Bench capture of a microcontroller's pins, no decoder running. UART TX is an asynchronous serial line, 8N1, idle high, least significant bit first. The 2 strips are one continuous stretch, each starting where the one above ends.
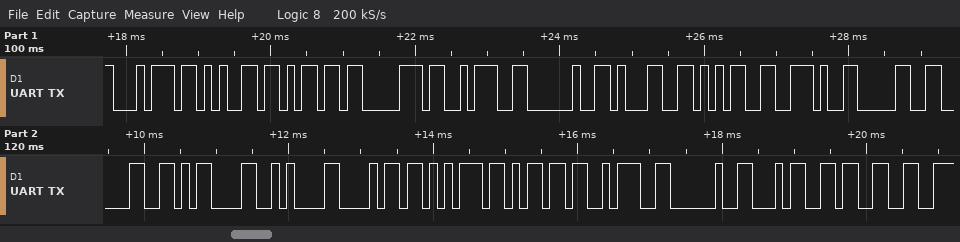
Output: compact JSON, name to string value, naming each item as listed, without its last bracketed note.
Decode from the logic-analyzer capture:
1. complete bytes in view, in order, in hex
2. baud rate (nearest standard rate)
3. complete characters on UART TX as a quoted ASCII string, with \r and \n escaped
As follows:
{"complete bytes in view, in order, in hex": "74 65 6D 70 3A 20 31 35 2E 30 30 0D 0A 68 75 6D 3A 20 34 33", "baud rate": "9600 baud", "complete characters on UART TX as a quoted ASCII string, with \\r and \\n escaped": "\"temp: 15.00\\r\\nhum: 43\""}
